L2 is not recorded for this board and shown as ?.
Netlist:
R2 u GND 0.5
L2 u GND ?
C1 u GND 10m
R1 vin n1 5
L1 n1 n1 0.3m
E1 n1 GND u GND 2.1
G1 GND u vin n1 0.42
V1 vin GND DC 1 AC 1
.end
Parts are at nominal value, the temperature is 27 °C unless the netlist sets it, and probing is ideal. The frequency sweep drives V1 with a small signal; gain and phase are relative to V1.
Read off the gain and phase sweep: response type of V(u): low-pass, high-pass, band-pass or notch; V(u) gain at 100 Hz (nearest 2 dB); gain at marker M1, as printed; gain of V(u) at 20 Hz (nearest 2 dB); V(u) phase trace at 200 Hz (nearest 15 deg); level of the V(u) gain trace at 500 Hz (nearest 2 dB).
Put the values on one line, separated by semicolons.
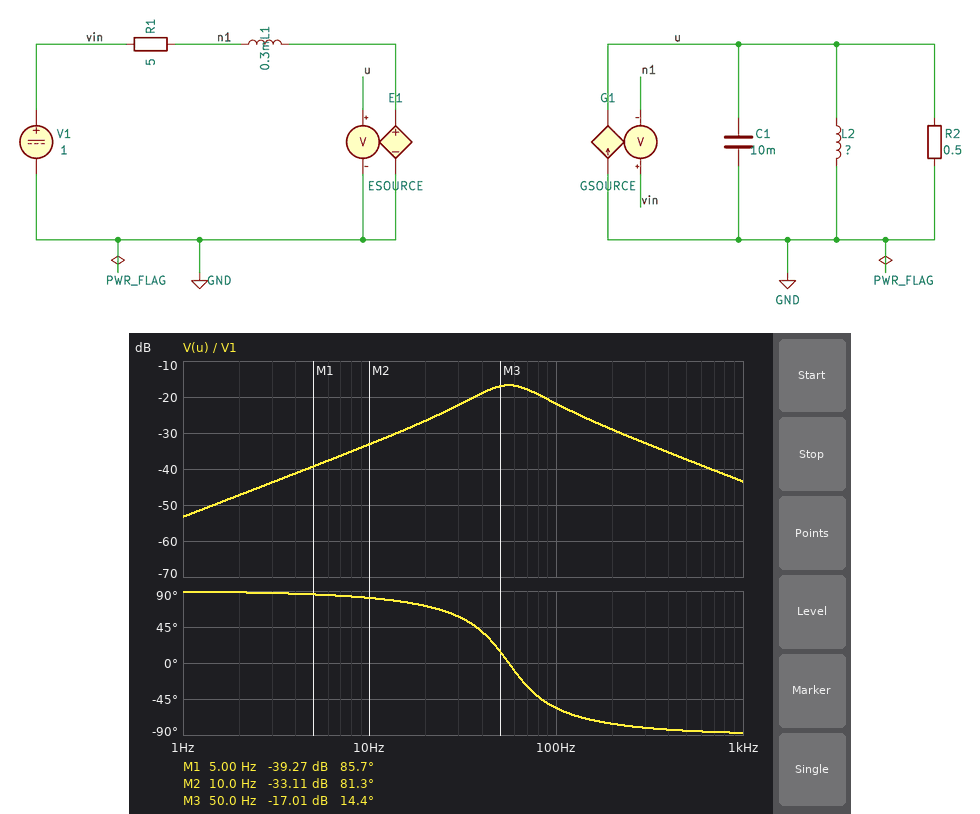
band-pass; -22 dB; -39.27 dB; -26 dB; -75 deg; -38 dB
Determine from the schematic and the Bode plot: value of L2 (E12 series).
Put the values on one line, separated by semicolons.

820 µH
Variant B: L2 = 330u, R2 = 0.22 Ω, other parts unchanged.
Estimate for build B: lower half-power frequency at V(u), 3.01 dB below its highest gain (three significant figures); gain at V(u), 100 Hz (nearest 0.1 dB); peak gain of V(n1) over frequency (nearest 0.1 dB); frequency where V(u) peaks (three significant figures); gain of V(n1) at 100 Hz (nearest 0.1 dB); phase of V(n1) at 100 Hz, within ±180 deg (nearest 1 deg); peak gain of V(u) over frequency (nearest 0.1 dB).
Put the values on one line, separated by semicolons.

54.5 Hz; -22.5 dB; -15.8 dB; 87.6 Hz; -16.1 dB; -15 deg; -22.2 dB
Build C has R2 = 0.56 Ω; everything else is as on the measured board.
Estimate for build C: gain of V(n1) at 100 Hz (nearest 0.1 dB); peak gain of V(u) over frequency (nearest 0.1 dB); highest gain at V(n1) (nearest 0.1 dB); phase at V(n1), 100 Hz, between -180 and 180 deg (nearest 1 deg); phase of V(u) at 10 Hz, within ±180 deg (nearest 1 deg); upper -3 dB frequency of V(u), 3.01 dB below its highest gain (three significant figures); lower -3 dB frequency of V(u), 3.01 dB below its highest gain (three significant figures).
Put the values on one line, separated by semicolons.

-15.2 dB; -16.1 dB; -9.6 dB; -58 deg; 82 deg; 80.7 Hz; 38.3 Hz
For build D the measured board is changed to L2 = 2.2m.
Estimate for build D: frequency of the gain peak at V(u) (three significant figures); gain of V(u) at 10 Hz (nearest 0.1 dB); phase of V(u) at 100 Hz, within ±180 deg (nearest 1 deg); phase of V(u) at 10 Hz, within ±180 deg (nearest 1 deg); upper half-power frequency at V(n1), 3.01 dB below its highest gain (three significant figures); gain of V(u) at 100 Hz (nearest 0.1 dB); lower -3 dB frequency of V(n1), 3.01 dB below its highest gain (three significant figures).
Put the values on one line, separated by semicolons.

33.9 Hz; -24.7 dB; -63 deg; 66 deg; 63.9 Hz; -23.5 dB; 18.0 Hz
